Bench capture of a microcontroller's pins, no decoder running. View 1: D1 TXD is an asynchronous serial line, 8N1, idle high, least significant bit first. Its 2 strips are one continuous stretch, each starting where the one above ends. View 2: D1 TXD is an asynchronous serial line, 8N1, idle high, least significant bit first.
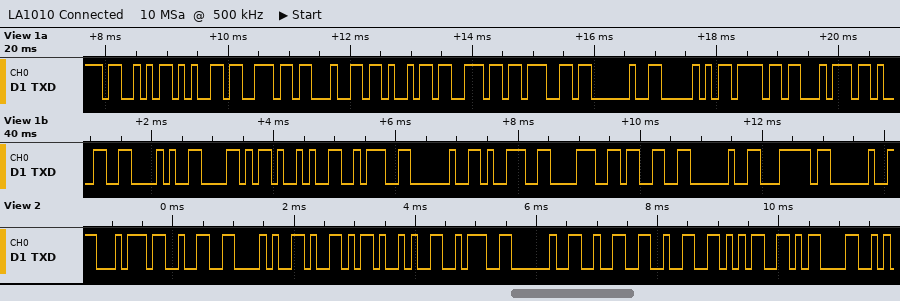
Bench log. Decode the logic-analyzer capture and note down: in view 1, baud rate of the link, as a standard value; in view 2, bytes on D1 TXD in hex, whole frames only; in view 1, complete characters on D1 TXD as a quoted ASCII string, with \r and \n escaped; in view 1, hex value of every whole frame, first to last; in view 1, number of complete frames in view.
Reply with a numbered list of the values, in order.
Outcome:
1. 9600 baud
2. 74 32 28 59 29 3A 20 32 32 35 0D
3. "Sending Pot1(X): 983 | "
4. 53 65 6E 64 69 6E 67 20 50 6F 74 31 28 58 29 3A 20 39 38 33 20 7C 20
5. 23
